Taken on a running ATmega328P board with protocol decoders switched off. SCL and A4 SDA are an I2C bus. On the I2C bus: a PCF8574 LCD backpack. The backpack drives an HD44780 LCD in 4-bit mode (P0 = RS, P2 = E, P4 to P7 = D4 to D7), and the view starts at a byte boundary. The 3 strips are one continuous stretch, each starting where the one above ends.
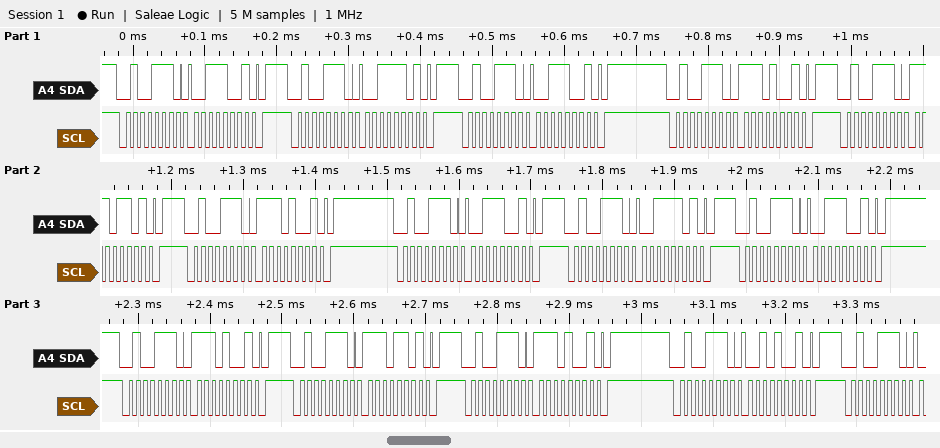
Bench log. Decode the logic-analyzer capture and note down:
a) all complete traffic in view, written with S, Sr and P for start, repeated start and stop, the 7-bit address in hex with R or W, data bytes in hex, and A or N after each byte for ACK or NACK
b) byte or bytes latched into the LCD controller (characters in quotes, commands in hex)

S 27W A 39 A P S 27W A 3D A P S 27W A 39 A P S 27W A E9 A P S 27W A ED A P S 27W A E9 A P S 27W A 39 A P S 27W A 3D A P S 27W A 39 A P S 27W A E9 A P S 27W A ED A P S 27W A E9 A P S 27W A 29 A P S 27W A
'>' '>'
